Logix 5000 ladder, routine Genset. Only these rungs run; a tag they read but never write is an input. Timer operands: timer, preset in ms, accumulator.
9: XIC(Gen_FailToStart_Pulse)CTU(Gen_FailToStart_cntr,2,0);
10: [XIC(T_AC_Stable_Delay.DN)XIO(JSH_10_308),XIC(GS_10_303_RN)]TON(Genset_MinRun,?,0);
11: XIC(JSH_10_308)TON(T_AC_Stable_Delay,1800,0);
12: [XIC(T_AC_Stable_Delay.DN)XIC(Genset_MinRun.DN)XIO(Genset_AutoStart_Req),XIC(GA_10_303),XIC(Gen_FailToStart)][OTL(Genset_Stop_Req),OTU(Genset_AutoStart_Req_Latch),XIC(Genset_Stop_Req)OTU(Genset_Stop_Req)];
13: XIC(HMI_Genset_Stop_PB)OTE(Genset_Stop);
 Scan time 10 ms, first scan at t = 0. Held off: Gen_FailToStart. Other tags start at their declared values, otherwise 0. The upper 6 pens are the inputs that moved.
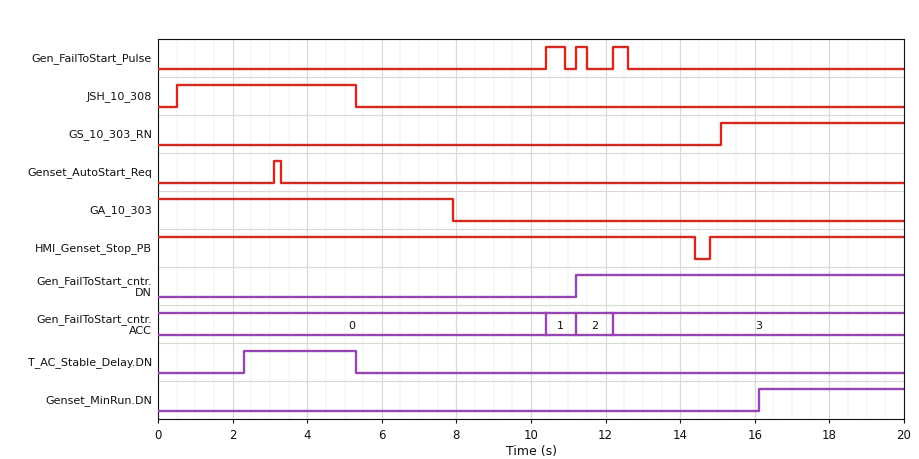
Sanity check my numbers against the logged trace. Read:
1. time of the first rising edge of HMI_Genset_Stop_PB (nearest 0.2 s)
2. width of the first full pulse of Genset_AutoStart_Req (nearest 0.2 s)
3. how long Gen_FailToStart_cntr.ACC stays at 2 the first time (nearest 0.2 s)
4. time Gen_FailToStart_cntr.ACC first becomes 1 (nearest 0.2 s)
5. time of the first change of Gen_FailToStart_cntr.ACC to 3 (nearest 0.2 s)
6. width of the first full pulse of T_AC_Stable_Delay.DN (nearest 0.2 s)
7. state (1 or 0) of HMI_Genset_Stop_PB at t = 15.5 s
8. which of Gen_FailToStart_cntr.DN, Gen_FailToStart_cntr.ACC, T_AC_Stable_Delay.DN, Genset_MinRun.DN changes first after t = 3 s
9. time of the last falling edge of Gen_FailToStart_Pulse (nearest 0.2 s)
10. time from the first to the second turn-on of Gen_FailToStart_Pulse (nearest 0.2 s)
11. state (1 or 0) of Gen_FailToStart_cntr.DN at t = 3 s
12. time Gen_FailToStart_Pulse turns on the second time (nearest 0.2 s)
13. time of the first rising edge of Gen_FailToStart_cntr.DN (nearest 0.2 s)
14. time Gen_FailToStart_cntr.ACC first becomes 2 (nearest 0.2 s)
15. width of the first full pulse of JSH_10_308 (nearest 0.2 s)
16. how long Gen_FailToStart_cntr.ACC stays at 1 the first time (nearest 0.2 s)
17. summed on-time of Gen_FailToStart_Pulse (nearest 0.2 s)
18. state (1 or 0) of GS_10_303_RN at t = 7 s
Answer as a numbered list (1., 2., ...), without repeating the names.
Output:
1. 14.8 s
2. 0.2 s
3. 1.0 s
4. 10.4 s
5. 12.2 s
6. 3.0 s
7. 1
8. T_AC_Stable_Delay.DN
9. 12.6 s
10. 0.8 s
11. 0
12. 11.2 s
13. 11.2 s
14. 11.2 s
15. 4.8 s
16. 0.8 s
17. 1.2 s
18. 0
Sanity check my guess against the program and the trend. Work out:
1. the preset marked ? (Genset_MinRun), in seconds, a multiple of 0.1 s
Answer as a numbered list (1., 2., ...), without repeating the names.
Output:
1. 1.0 s
